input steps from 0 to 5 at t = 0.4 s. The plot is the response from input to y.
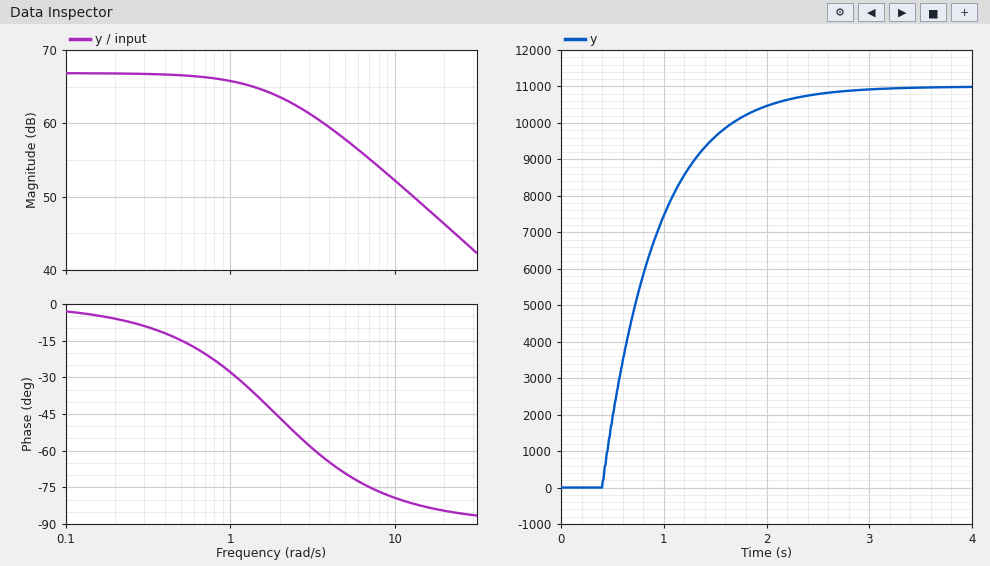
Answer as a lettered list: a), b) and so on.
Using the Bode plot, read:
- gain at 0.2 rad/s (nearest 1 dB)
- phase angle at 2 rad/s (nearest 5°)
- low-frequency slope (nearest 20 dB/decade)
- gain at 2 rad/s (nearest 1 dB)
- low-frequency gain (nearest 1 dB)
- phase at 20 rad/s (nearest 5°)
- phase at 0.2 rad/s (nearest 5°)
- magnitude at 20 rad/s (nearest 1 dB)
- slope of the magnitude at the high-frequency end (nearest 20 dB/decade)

a) 67 dB
b) -45°
c) 0 dB/decade
d) 64 dB
e) 67 dB
f) -85°
g) -5°
h) 46 dB
i) -20 dB/decade
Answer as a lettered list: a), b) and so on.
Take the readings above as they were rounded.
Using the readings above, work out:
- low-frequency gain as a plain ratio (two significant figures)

a) 2200
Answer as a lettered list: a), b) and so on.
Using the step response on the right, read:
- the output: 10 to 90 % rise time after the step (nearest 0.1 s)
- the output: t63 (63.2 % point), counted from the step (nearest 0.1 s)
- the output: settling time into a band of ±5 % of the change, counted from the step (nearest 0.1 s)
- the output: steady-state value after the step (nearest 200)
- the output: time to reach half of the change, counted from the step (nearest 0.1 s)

a) 1.2 s
b) 0.5 s
c) 1.6 s
d) 11000
e) 0.4 s
